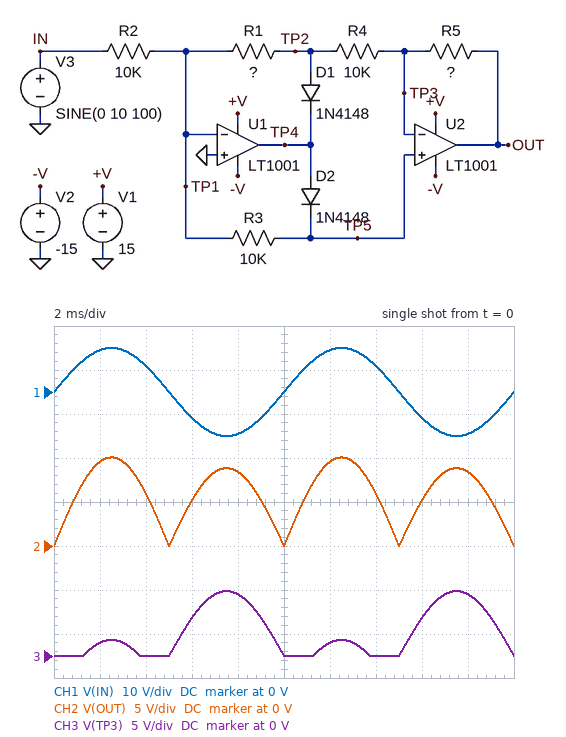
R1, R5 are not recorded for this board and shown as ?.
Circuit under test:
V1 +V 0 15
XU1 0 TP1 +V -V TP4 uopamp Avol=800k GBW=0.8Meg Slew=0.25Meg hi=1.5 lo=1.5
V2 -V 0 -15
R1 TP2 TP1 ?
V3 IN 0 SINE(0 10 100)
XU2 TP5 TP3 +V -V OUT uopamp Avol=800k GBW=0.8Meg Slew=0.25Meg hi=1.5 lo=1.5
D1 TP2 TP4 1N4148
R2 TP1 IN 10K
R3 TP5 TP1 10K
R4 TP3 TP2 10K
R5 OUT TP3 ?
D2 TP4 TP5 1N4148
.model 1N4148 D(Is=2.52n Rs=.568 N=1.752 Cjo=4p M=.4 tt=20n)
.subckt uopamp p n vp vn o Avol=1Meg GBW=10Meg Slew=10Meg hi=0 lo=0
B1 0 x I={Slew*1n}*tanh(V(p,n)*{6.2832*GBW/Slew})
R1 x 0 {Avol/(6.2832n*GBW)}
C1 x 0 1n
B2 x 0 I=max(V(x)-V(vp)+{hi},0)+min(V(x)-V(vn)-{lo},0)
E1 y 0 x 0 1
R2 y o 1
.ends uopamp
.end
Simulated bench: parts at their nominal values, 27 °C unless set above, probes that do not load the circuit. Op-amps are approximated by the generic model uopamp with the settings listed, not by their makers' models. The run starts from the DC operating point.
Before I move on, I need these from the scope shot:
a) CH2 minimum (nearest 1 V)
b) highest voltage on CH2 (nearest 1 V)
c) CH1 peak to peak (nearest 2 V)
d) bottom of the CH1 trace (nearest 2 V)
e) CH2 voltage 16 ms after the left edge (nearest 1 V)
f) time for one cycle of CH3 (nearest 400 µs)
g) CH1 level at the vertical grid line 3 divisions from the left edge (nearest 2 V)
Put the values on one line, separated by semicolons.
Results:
0 V; 10 V; 20 V; -10 V; 5 V; 10.0 ms; -6 V
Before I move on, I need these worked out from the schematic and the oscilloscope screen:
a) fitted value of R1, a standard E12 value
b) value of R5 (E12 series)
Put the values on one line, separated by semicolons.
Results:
18 kΩ; 5.6 kΩ
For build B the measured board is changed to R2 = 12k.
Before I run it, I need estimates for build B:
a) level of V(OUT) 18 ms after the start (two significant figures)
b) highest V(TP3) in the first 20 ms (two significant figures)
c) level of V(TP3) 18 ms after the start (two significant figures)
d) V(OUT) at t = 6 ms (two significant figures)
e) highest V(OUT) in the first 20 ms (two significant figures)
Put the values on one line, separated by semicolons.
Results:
7.0 V; 6.1 V; 5.8 V; 4.3 V; 8.5 V
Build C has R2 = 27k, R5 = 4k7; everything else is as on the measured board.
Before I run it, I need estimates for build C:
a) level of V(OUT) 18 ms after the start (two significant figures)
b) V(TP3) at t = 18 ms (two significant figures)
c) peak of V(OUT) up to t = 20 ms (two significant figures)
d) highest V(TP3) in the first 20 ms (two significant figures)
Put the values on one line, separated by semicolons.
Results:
3.0 V; 2.6 V; 3.2 V; 2.7 V
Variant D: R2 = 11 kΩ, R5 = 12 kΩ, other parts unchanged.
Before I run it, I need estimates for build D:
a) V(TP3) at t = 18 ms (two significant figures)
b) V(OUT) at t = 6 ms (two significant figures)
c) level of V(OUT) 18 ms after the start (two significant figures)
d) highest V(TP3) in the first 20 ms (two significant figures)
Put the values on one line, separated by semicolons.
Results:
6.4 V; 5.6 V; 9.1 V; 6.7 V
